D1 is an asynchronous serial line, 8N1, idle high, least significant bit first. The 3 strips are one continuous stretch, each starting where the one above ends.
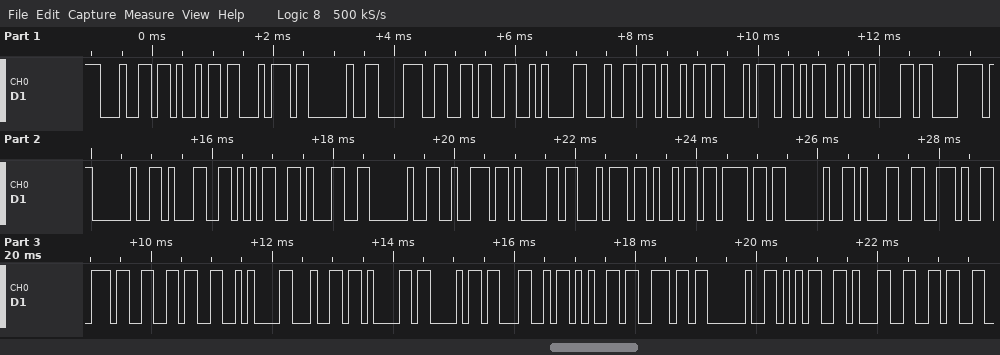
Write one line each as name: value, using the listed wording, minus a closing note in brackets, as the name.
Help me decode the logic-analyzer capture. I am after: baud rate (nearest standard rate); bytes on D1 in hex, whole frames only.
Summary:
baud rate: 9600 baud
bytes on D1 in hex, whole frames only: 64 69 74 20 38 36 0A 64 69 74 4D 61 78 20 31 35 31 20 72 61 74 69 6F 20 31 2E 37 36 0A 64 61 68 4C 65 6E 20 35 31 36
